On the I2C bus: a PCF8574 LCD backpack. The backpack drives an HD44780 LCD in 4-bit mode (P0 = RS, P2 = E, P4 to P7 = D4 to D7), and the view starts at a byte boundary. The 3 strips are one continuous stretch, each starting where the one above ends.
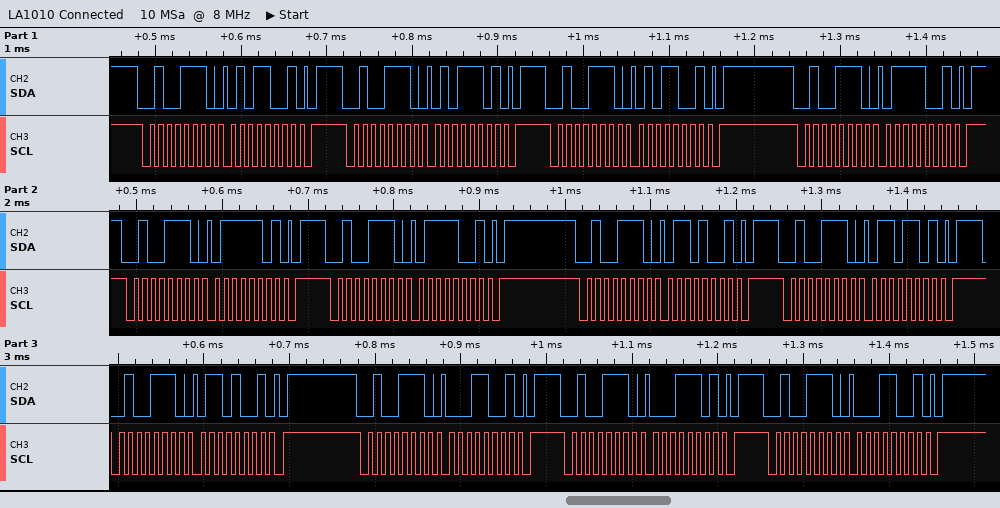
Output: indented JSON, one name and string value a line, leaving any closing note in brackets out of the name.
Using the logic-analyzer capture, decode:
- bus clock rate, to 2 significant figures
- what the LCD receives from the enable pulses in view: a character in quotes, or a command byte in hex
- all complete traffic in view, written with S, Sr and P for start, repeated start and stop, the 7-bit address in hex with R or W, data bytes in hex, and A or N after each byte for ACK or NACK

{
  "bus clock rate, to 2 significant figures": "100 kHz",
  "what the LCD receives from the enable pulses in view: a character in quotes, or a command byte in hex": "'W' 'a'",
  "all complete traffic in view, written with S, Sr and P for start, repeated start and stop, the 7-bit address in hex with R or W, data bytes in hex, and A or N after each byte for ACK or NACK": "S 27W A 59 A P S 27W A 5D A P S 27W A 59 A P S 27W A 79 A P S 27W A 7D A P S 27W A 79 A P S 27W A 69 A P S 27W A 6D A P S 27W A 69 A P S 27W A 19 A P S 27W A 1D A P S 27W A 19 A P"
}
